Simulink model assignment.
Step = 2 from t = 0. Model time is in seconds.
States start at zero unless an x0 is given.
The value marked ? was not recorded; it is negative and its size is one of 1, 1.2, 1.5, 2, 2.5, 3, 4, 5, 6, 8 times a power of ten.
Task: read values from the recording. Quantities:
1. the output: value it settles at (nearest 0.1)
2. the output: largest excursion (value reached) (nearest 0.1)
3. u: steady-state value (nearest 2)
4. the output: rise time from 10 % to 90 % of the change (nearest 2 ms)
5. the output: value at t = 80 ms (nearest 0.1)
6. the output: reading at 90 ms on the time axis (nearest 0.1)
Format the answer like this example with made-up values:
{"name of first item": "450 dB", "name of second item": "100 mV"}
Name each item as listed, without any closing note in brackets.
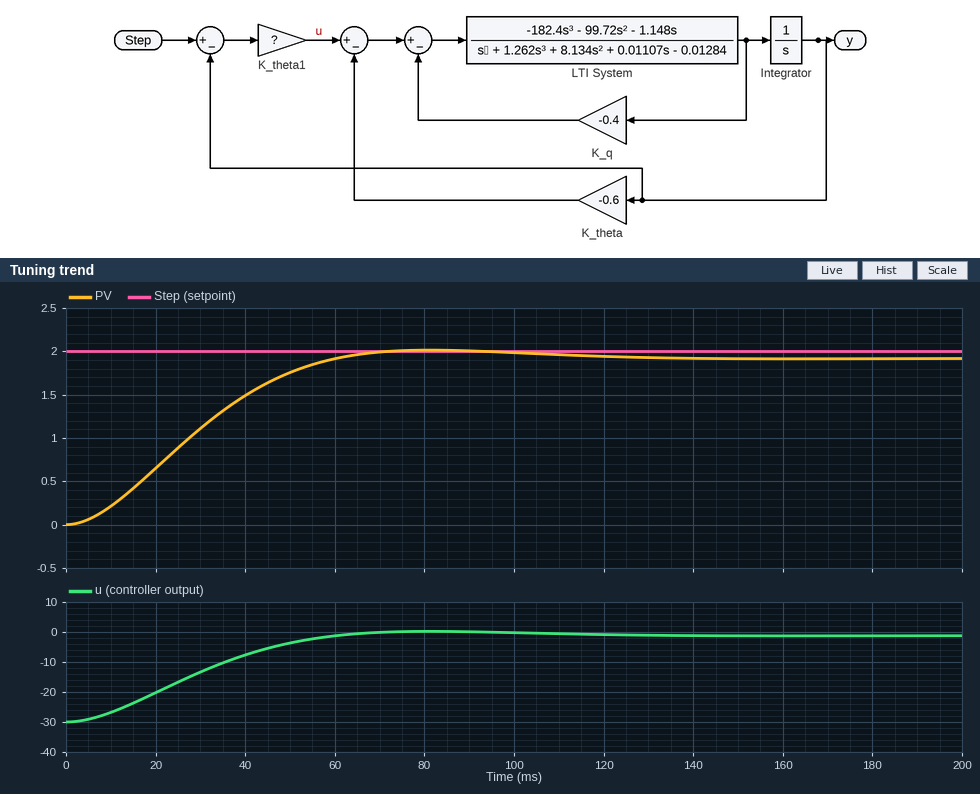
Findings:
{"the output: value it settles at": "1.9", "the output: largest excursion (value reached)": "2.0", "u: steady-state value": "-2", "the output: rise time from 10 % to 90 % of the change": "40 ms", "the output: value at t = 80 ms": "2.0", "the output: reading at 90 ms on the time axis": "2.0"}
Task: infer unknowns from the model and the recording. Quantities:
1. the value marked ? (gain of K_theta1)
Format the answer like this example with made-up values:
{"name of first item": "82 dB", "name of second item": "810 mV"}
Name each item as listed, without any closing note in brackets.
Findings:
{"the value marked ?": "-15"}
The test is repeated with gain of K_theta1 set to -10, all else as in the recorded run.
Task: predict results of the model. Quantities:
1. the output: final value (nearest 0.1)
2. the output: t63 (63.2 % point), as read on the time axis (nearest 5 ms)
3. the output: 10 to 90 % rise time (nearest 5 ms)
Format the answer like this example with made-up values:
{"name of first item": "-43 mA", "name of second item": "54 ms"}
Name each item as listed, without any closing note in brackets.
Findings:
{"the output: final value": "1.9", "the output: t63 (63.2 % point), as read on the time axis": "45 ms", "the output: 10 to 90 % rise time": "60 ms"}
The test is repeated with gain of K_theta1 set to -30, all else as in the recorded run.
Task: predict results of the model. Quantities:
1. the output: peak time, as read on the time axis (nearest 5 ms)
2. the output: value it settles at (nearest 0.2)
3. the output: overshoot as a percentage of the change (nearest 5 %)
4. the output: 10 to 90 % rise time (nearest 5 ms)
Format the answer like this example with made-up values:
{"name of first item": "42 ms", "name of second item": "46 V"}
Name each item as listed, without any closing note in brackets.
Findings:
{"the output: peak time, as read on the time axis": "50 ms", "the output: value it settles at": "2.0", "the output: overshoot as a percentage of the change": "15 %", "the output: 10 to 90 % rise time": "20 ms"}
